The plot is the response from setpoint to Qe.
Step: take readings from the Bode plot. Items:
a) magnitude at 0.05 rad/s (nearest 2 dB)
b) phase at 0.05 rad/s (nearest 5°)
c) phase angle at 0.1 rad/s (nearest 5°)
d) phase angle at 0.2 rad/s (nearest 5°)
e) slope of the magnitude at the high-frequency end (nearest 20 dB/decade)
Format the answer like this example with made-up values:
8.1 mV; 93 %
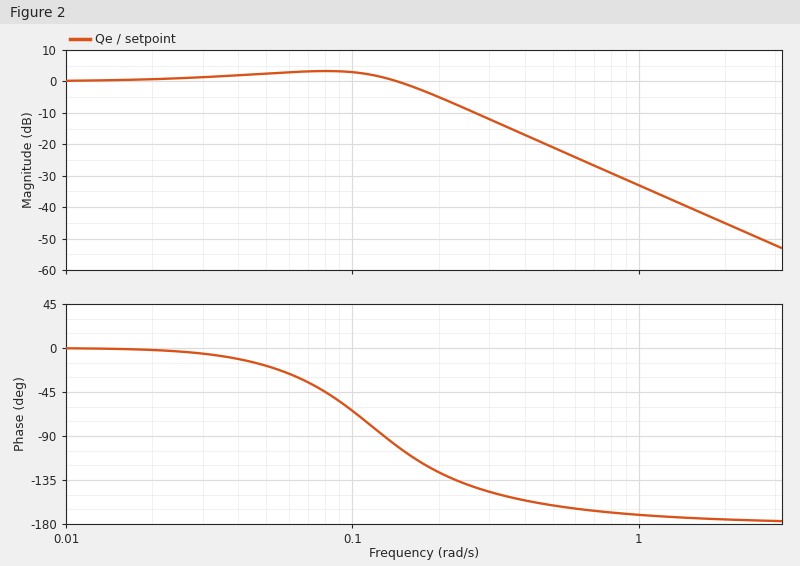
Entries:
2 dB; -20°; -65°; -125°; -40 dB/decade
